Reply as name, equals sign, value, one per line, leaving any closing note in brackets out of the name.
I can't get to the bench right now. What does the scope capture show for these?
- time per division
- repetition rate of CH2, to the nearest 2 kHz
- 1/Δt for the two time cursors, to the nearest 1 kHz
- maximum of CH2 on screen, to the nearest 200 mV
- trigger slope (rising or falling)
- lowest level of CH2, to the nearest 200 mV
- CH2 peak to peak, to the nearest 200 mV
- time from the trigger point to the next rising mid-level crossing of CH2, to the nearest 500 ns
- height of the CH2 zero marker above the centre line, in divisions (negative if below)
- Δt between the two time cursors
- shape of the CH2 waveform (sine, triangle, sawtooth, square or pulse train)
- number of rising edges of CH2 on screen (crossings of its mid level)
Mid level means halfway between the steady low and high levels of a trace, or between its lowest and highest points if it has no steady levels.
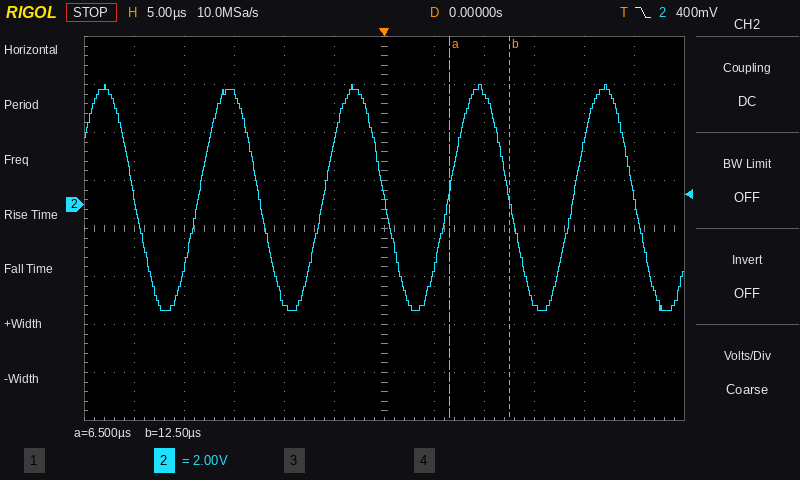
time per division = 5 µs
repetition rate of CH2, to the nearest 2 kHz = 80 kHz
1/Δt for the two time cursors, to the nearest 1 kHz = 167 kHz
maximum of CH2 on screen, to the nearest 200 mV = 5.0 V
trigger slope = falling
lowest level of CH2, to the nearest 200 mV = -4.4 V
CH2 peak to peak, to the nearest 200 mV = 9.4 V
time from the trigger point to the next rising mid-level crossing of CH2, to the nearest 500 ns = 6.5 µs
height of the CH2 zero marker above the centre line, in divisions = +0.5 div
Δt between the two time cursors = 6.0 µs
shape of the CH2 waveform = sine
number of rising edges of CH2 on screen = 4
